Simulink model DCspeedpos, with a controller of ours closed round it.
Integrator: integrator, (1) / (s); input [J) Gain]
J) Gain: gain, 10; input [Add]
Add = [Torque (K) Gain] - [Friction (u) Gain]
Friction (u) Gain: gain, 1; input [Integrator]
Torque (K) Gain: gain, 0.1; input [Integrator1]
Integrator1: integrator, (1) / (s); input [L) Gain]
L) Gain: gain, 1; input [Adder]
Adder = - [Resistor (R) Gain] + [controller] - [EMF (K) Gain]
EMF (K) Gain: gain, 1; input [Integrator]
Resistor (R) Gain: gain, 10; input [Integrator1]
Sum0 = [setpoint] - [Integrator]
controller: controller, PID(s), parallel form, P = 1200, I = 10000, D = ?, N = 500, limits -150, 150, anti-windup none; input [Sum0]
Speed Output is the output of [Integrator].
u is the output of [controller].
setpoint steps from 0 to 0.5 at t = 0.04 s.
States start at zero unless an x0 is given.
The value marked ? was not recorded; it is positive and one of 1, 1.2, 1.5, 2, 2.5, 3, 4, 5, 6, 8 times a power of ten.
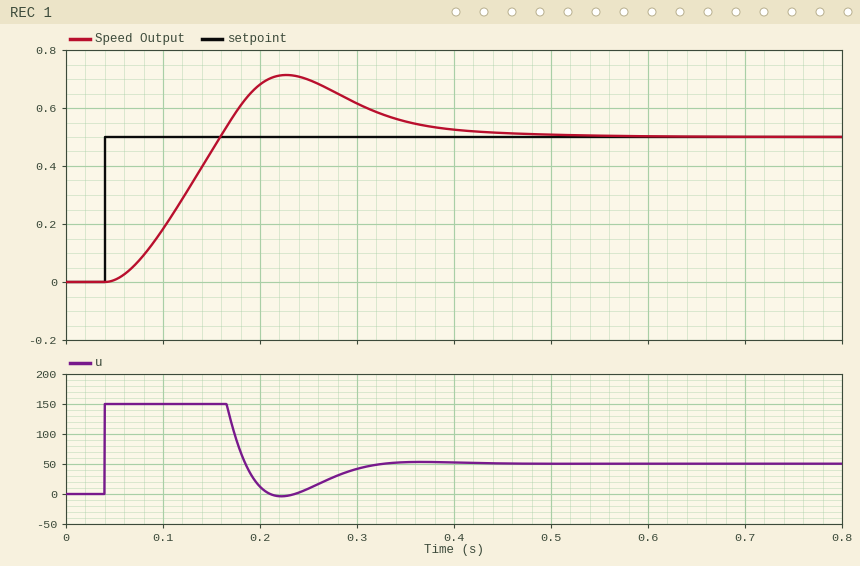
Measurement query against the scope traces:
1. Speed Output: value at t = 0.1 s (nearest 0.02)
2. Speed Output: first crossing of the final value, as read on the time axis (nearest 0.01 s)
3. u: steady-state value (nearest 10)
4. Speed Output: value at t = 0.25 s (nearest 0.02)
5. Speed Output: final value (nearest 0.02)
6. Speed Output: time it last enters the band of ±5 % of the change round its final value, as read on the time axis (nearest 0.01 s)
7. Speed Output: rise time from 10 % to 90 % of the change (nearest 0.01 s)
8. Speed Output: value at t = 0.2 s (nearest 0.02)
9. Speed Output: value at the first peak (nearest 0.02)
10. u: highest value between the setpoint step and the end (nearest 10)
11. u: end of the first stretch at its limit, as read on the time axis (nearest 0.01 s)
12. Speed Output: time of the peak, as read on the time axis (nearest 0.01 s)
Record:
0.18
0.16 s
50
0.70
0.50
0.40 s
0.08 s
0.68
0.72
150
0.17 s
0.23 s
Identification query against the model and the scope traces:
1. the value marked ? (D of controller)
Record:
30
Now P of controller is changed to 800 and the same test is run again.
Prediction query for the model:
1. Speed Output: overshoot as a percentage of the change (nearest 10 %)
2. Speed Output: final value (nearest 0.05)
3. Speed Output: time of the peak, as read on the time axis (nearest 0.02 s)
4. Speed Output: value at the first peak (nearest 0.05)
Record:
50 %
0.50
0.24 s
0.75
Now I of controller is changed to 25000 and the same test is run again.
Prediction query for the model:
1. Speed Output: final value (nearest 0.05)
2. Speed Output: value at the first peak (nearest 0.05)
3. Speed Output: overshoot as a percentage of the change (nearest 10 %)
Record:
0.50
0.90
80 %
